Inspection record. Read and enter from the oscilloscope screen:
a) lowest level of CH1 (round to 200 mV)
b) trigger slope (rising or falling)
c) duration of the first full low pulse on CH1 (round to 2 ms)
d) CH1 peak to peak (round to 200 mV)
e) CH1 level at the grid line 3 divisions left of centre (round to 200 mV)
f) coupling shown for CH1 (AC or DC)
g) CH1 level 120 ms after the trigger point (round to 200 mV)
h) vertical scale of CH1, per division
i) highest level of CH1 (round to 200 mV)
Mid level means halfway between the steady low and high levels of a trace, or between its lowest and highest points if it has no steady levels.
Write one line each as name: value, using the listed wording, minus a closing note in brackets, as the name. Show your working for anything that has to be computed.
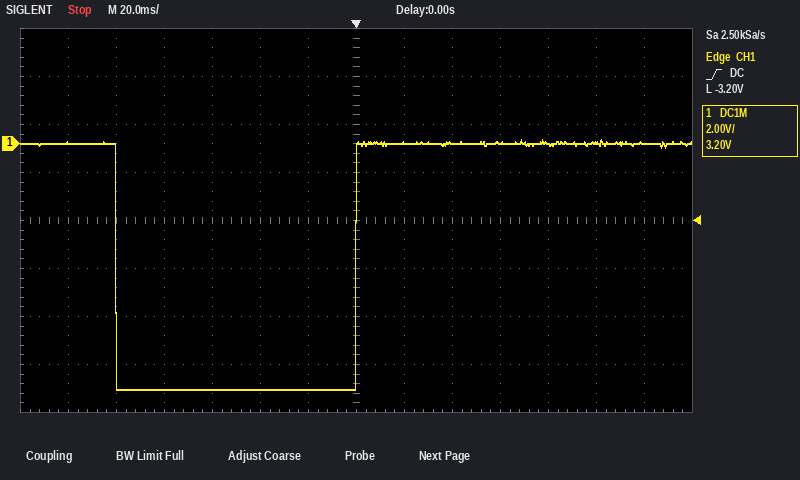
lowest level of CH1: -10.2 V
trigger slope: rising
duration of the first full low pulse on CH1: 100 ms
CH1 peak to peak: 200 mV − (-10.2 V) = 10.4 V
CH1 level at the grid line 3 divisions left of centre: -10.2 V
coupling shown for CH1: DC
CH1 level 120 ms after the trigger point: 0.0 V
vertical scale of CH1, per division: 2 V
highest level of CH1: 200 mV
